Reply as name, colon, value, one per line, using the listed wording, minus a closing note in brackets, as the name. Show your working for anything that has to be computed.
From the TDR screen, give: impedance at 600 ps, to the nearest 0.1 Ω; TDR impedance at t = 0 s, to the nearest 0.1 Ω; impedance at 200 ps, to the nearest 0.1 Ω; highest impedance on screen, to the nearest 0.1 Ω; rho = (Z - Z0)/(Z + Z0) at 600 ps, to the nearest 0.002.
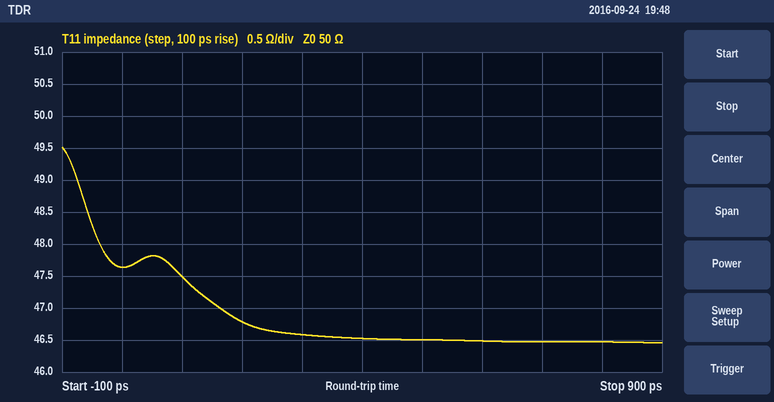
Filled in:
impedance at 600 ps, to the nearest 0.1 Ω: 46.5 Ω
TDR impedance at t = 0 s, to the nearest 0.1 Ω: 47.6 Ω
impedance at 200 ps, to the nearest 0.1 Ω: 46.8 Ω
highest impedance on screen, to the nearest 0.1 Ω: 49.5 Ω
rho = (Z - Z0)/(Z + Z0) at 600 ps, to the nearest 0.002: (46.5 − 50)/(46.5 + 50) ≈ -0.036
